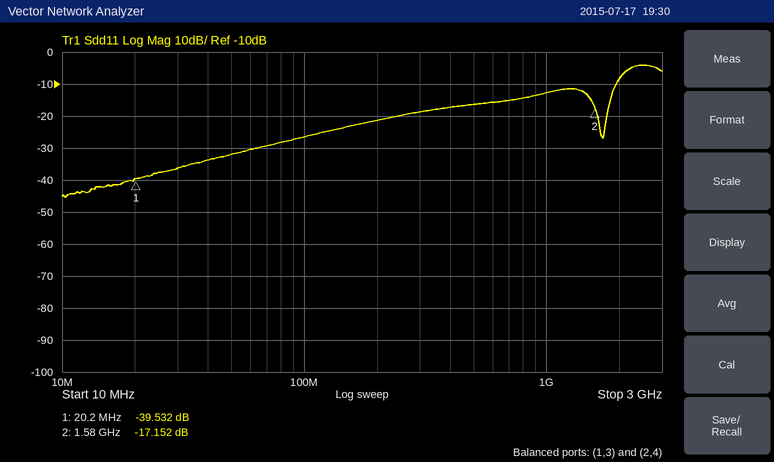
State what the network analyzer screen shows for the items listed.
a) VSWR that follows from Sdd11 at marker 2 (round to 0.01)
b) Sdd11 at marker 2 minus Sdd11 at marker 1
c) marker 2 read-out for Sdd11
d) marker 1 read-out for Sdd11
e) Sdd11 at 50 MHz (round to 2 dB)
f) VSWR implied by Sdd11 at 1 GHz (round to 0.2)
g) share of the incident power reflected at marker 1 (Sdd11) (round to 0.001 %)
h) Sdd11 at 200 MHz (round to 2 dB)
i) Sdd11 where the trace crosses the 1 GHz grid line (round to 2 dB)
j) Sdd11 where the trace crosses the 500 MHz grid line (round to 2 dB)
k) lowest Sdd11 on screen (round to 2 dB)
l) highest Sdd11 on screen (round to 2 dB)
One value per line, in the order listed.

1.32
22.380 dB
-17.152 dB
-39.532 dB
-32 dB
1.6
0.011 %
-22 dB
-12 dB
-16 dB
-46 dB
-4 dB
